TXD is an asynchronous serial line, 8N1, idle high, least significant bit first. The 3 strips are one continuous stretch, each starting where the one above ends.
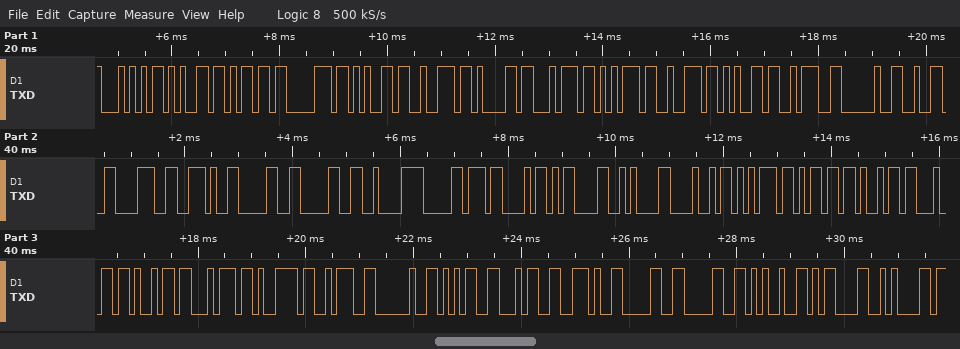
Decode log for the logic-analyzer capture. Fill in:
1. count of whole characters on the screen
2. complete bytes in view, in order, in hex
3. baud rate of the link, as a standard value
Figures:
41
54 65 6D 70 65 72 61 74 75 72 65 3A 20 32 38 2E 30 30 C2 B0 43 0D 0A 48 75 6D 69 64 69 74 79 3A 20 35 34 2E 30 30 25 0D 0A
9600 baud
